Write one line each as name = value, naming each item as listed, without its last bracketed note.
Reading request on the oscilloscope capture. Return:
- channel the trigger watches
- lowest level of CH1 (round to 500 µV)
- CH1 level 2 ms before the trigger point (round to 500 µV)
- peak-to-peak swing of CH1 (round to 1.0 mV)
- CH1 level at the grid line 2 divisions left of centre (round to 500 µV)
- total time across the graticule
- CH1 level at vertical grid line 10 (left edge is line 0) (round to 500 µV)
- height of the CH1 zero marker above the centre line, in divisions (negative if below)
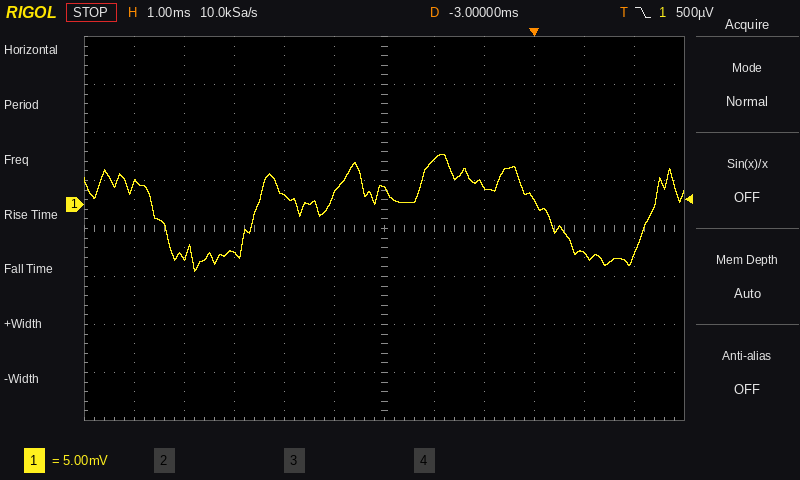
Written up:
channel the trigger watches = CH1
lowest level of CH1 = -7.0 mV
CH1 level 2 ms before the trigger point = 4.5 mV
peak-to-peak swing of CH1 = 12.0 mV
CH1 level at the grid line 2 divisions left of centre = 1.0 mV
total time across the graticule = 12 ms
CH1 level at vertical grid line 10 (left edge is line 0) = -5.0 mV
height of the CH1 zero marker above the centre line, in divisions = +0.5 div
